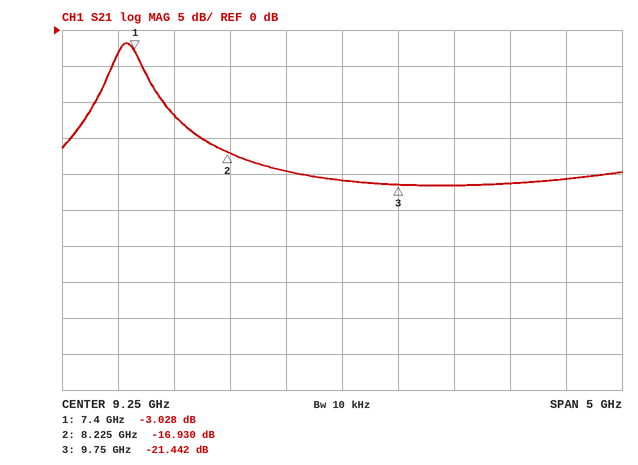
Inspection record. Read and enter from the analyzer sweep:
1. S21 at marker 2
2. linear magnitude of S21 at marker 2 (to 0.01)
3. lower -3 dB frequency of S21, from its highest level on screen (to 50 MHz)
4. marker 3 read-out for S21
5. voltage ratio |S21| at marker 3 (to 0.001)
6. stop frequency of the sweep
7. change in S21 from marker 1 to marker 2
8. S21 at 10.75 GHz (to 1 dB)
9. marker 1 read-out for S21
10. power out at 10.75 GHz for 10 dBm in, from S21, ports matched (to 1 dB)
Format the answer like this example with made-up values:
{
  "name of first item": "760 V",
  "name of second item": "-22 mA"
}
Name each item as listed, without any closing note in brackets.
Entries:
{
  "S21 at marker 2": "-16.930 dB",
  "linear magnitude of S21 at marker 2": "0.14",
  "lower -3 dB frequency of S21, from its highest level on screen": "7.20 GHz",
  "marker 3 read-out for S21": "-21.442 dB",
  "voltage ratio |S21| at marker 3": "0.085",
  "stop frequency of the sweep": "11.75 GHz",
  "change in S21 from marker 1 to marker 2": "-13.902 dB",
  "S21 at 10.75 GHz": "-21 dB",
  "marker 1 read-out for S21": "-3.028 dB",
  "power out at 10.75 GHz for 10 dBm in, from S21, ports matched": "-11 dBm"
}
